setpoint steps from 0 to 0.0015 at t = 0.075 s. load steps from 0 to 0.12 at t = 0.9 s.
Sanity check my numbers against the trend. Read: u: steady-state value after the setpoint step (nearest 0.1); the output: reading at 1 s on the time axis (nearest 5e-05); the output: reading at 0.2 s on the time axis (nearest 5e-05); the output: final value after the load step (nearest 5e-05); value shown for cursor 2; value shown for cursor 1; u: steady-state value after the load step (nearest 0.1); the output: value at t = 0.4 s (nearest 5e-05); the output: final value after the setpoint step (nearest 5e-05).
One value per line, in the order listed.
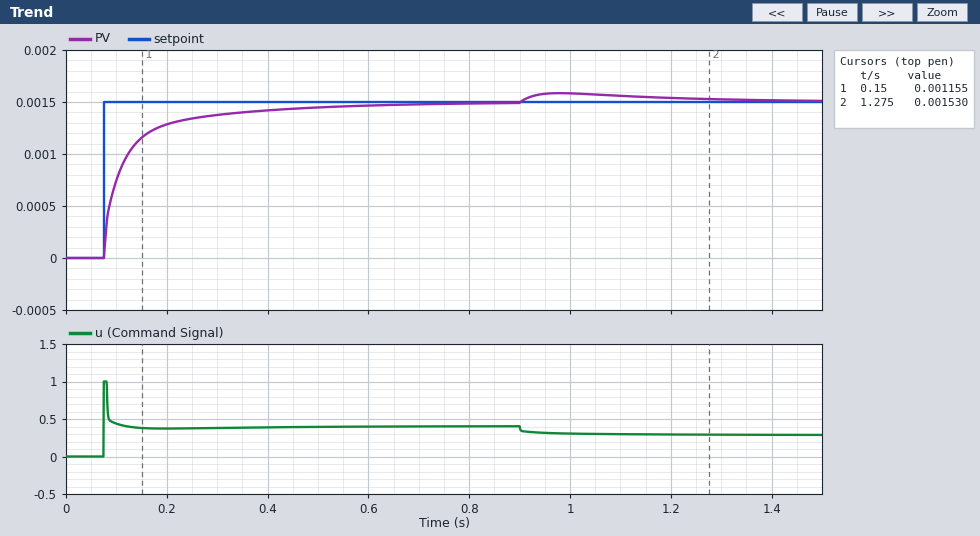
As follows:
0.4
0.00160
0.00130
0.00150
0.001530
0.001155
0.3
0.00140
0.00150
